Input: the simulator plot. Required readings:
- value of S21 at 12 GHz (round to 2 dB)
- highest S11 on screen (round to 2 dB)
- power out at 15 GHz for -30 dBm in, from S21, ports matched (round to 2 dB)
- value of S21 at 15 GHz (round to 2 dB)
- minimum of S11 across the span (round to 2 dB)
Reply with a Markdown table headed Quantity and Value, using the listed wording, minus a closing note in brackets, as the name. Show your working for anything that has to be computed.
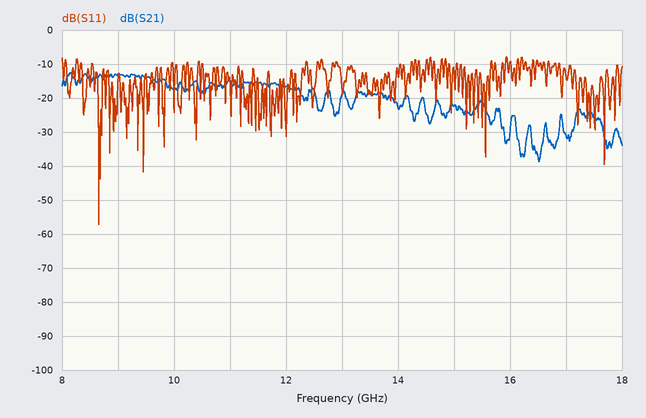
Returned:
| Quantity | Value |
|---|---|
| value of S21 at 12 GHz | -16 dB |
| highest S11 on screen | -8 dB |
| power out at 15 GHz for -30 dBm in, from S21, ports matched | -30 dBm + (-22 dB) = -52 dBm |
| value of S21 at 15 GHz | -22 dB |
| minimum of S11 across the span | -58 dB |
